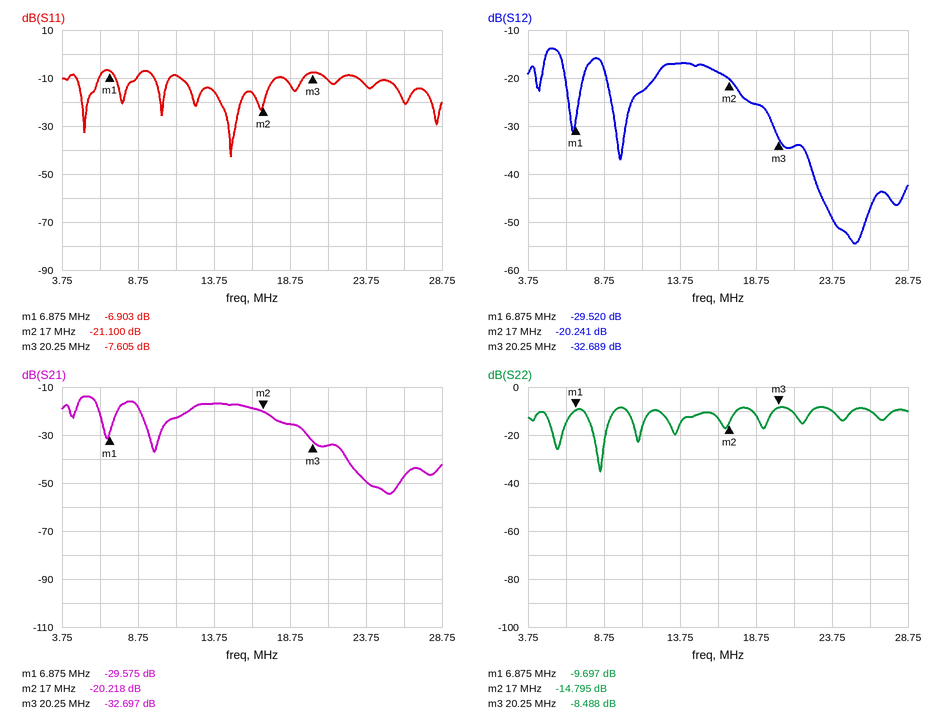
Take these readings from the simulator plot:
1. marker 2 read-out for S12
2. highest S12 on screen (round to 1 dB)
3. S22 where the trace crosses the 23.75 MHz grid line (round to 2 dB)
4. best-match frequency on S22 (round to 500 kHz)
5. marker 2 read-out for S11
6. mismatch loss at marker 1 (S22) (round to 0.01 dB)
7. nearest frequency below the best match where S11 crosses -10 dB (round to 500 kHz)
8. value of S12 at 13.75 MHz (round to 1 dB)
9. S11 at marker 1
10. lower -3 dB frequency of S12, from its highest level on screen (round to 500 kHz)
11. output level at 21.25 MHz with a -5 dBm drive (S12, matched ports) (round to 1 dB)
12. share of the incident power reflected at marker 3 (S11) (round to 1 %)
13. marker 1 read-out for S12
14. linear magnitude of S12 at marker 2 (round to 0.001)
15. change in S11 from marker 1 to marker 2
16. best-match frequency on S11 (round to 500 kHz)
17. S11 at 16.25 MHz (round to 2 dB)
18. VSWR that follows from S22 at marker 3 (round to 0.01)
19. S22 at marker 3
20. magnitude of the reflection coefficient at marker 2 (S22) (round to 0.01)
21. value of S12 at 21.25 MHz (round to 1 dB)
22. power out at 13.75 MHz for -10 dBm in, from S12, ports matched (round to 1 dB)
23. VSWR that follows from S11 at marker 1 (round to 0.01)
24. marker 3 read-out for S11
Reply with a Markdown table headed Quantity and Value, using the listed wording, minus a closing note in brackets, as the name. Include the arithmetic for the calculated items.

| Quantity | Value |
|---|---|
| marker 2 read-out for S12 | -20.241 dB |
| highest S12 on screen | -14 dB |
| S22 where the trace crosses the 23.75 MHz grid line | -10 dB |
| best-match frequency on S22 | 8.5 MHz |
| marker 2 read-out for S11 | -21.100 dB |
| mismatch loss at marker 1 (S22) | −10 log10(1 − 10^(-9.697/10)) ≈ 0.49 dB |
| nearest frequency below the best match where S11 crosses -10 dB | 11.5 MHz |
| value of S12 at 13.75 MHz | -17 dB |
| S11 at marker 1 | -6.903 dB |
| lower -3 dB frequency of S12, from its highest level on screen | 5.0 MHz |
| output level at 21.25 MHz with a -5 dBm drive (S12, matched ports) | -5 dBm + (-34 dB) = -39 dBm |
| share of the incident power reflected at marker 3 (S11) | 10^(-7.605/10) ≈ 17 % |
| marker 1 read-out for S12 | -29.520 dB |
| linear magnitude of S12 at marker 2 | 10^(-20.241/20) ≈ 0.097 |
| change in S11 from marker 1 to marker 2 | -21.1 − (-6.903) = -14.197 dB |
| best-match frequency on S11 | 15.0 MHz |
| S11 at 16.25 MHz | -16 dB |
| VSWR that follows from S22 at marker 3 | (1 + 0.3764)/(1 − 0.3764) ≈ 2.21 |
| S22 at marker 3 | -8.488 dB |
| magnitude of the reflection coefficient at marker 2 (S22) | 10^(-14.795/20) ≈ 0.18 |
| value of S12 at 21.25 MHz | -34 dB |
| power out at 13.75 MHz for -10 dBm in, from S12, ports matched | -10 dBm + (-17 dB) = -27 dBm |
| VSWR that follows from S11 at marker 1 | (1 + 0.4517)/(1 − 0.4517) ≈ 2.65 |
| marker 3 read-out for S11 | -7.605 dB |
